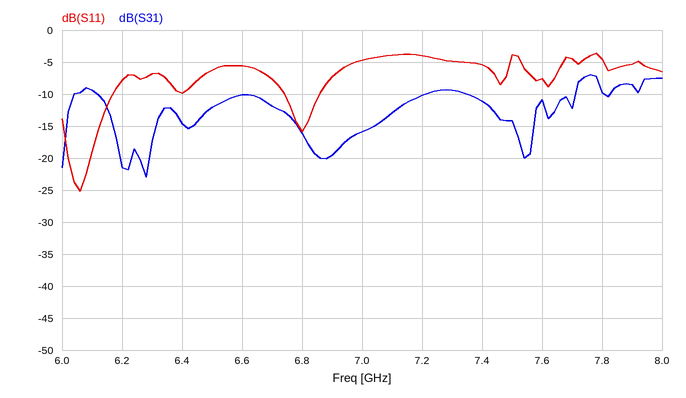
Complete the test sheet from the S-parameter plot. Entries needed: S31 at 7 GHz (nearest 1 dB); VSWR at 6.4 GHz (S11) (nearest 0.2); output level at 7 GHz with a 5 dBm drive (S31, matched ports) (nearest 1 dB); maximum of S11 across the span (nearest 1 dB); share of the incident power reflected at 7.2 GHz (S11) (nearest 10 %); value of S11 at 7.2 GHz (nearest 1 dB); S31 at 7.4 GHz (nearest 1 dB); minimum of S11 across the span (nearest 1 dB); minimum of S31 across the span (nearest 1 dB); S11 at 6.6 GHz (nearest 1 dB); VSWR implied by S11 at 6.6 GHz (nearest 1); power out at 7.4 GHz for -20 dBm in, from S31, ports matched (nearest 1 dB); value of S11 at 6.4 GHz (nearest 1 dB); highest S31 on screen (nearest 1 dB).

-16 dB
2.0
-11 dBm
-4 dB
40 %
-4 dB
-11 dB
-25 dB
-23 dB
-6 dB
3
-31 dBm
-10 dB
-7 dB
